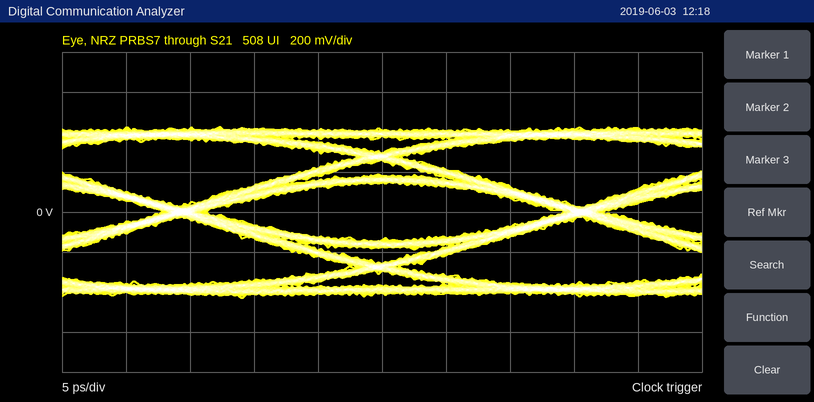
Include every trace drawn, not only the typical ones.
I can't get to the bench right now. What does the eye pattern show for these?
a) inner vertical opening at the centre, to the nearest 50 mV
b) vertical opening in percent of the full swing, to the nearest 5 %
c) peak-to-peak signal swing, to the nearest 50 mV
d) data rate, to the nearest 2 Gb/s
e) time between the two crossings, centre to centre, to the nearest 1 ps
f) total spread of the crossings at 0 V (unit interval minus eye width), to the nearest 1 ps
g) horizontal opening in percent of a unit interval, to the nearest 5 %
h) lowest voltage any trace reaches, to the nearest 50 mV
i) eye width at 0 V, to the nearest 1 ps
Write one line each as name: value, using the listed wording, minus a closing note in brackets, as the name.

inner vertical opening at the centre, to the nearest 50 mV: 300 mV
vertical opening in percent of the full swing, to the nearest 5 %: 35 %
peak-to-peak signal swing, to the nearest 50 mV: 850 mV
data rate, to the nearest 2 Gb/s: 32 Gb/s
time between the two crossings, centre to centre, to the nearest 1 ps: 31 ps
total spread of the crossings at 0 V (unit interval minus eye width), to the nearest 1 ps: 3 ps
horizontal opening in percent of a unit interval, to the nearest 5 %: 90 %
lowest voltage any trace reaches, to the nearest 50 mV: -450 mV
eye width at 0 V, to the nearest 1 ps: 28 ps
